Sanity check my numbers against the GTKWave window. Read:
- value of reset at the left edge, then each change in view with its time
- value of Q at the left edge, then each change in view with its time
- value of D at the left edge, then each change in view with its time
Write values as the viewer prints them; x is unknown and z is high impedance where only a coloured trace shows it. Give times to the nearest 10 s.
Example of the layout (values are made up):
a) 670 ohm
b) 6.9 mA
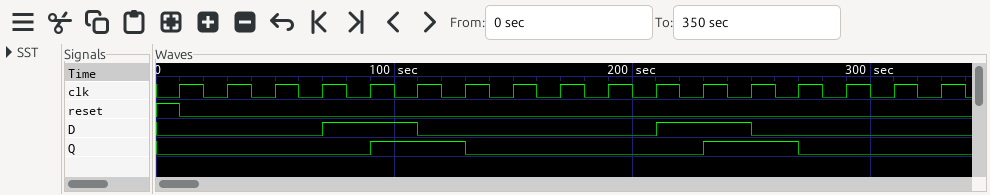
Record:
a) 1, 0 at 10 s
b) 0, 1 at 90 s, 0 at 130 s, 1 at 230 s, 0 at 270 s
c) 0, 1 at 70 s, 0 at 110 s, 1 at 210 s, 0 at 250 s
